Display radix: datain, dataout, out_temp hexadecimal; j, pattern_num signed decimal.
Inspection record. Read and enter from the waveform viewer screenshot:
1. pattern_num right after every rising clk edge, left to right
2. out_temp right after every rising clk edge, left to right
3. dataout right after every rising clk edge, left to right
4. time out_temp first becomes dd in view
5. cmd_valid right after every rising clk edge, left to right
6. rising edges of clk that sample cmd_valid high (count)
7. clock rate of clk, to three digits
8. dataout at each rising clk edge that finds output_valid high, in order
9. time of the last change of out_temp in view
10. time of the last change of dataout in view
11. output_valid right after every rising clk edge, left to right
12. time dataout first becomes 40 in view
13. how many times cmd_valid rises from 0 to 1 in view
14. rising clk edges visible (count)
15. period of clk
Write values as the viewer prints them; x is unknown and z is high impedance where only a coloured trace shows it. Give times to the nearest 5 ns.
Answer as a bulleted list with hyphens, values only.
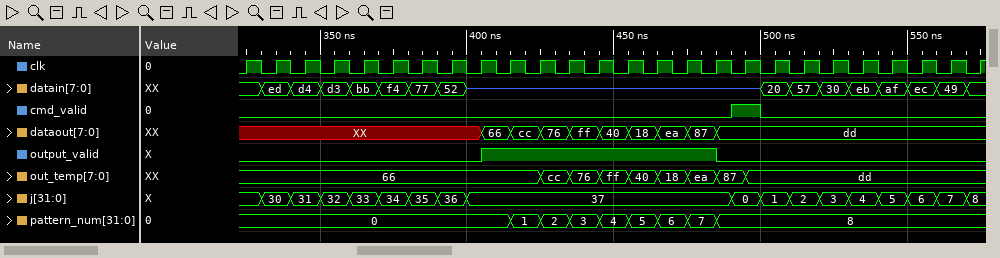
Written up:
- 0, 0, 0, 0, 0, 0, 0, 0, 0, 1, 2, 3, 4, 5, 6, 7, 8, 8, 8, 8, 8, 8, 8, 8, 8, 8
- 66, 66, 66, 66, 66, 66, 66, 66, 66, 66, cc, 76, ff, 40, 18, ea, 87, dd, dd, dd, dd, dd, dd, dd, dd, dd
- XX, XX, XX, XX, XX, XX, XX, XX, 66, cc, 76, ff, 40, 18, ea, 87, dd, dd, dd, dd, dd, dd, dd, dd, dd, dd
- 495 ns
- 0 0 0 0 0 0 0 0 0 0 0 0 0 0 0 0 0 1 0 0 0 0 0 0 0 0
- 1
- 100 MHz
- 66, cc, 76, ff, 40, 18, ea, 87
- 495 ns
- 485 ns
- 0 0 0 0 0 0 0 0 1 1 1 1 1 1 1 1 0 0 0 0 0 0 0 0 0 0
- 445 ns
- 1
- 26
- 10 ns
